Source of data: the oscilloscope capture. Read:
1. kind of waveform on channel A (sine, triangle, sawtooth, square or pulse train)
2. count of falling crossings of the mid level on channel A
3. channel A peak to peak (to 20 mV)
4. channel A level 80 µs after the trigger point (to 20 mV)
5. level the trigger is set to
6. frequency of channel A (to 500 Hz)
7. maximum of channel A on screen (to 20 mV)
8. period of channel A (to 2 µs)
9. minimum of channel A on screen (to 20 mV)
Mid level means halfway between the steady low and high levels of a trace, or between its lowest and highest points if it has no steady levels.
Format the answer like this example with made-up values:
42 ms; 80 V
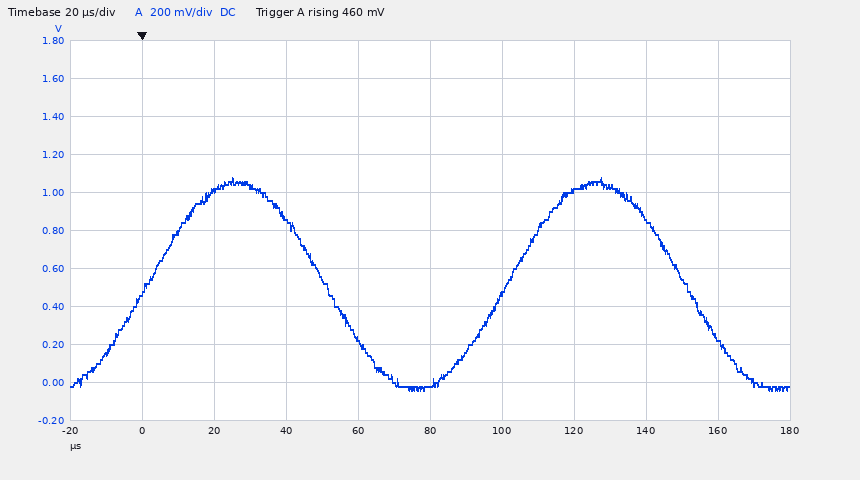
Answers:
sine; 2; 1.12 V; -20 mV; 460 mV; 10.0 kHz; 1.08 V; 100 µs; -40 mV
